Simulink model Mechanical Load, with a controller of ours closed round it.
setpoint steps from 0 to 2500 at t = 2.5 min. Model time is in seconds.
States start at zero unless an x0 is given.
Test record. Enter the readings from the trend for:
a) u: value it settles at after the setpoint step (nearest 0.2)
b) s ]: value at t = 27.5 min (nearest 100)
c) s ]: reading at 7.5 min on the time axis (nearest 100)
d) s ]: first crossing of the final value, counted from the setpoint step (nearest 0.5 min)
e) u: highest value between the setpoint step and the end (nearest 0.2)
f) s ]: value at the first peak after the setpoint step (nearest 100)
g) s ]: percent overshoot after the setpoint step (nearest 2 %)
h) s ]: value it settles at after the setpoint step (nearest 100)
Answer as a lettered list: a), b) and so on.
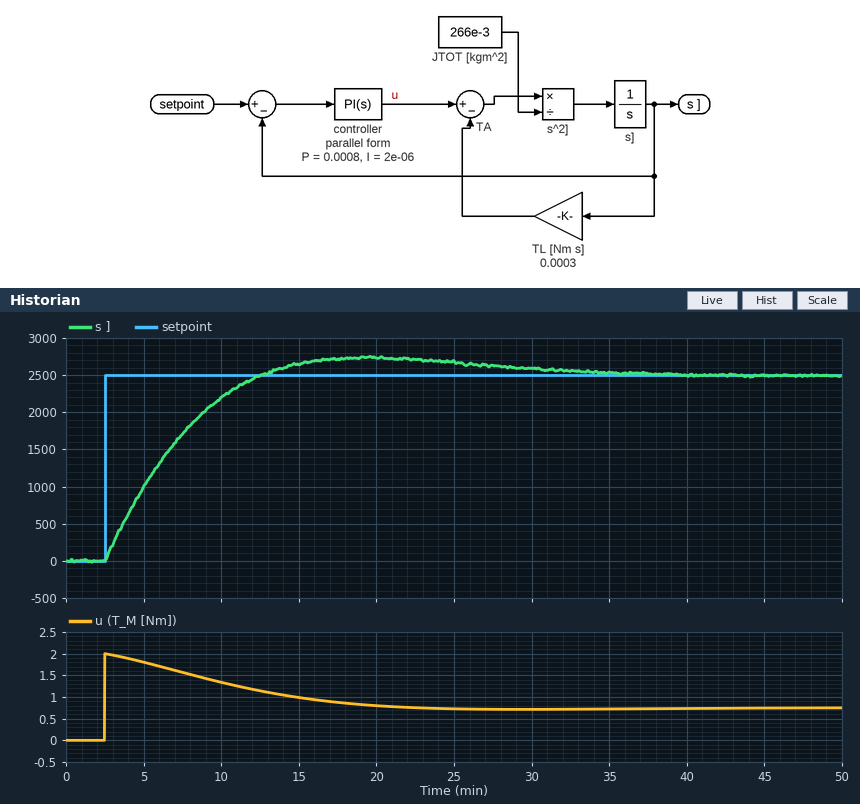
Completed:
a) 0.8
b) 2600
c) 1700
d) 10.0 min
e) 2.0
f) 2700
g) 10 %
h) 2500
